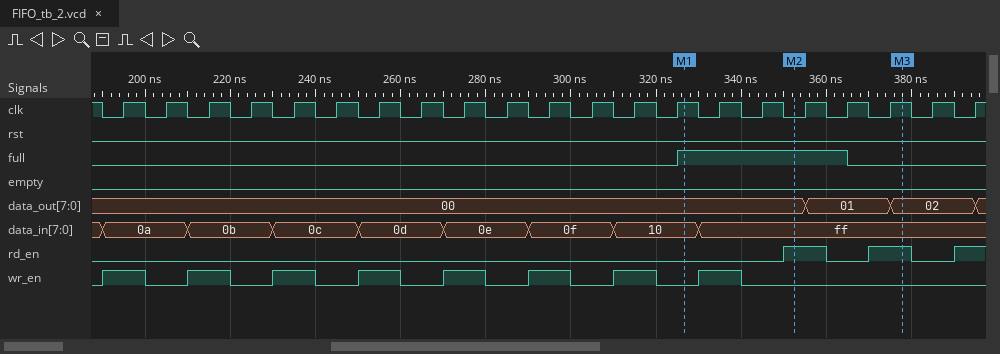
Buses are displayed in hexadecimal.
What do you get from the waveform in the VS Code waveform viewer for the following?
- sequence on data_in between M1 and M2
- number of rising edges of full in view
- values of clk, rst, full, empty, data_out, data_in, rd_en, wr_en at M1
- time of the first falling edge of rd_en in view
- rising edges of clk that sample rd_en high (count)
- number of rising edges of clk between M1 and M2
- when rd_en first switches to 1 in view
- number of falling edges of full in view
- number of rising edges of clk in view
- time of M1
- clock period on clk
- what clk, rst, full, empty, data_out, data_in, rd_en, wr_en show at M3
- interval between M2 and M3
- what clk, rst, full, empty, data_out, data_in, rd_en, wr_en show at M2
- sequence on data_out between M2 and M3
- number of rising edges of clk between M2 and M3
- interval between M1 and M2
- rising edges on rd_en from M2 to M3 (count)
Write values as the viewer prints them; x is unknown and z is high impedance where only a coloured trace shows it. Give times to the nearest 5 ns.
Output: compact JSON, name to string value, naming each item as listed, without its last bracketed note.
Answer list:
{"sequence on data_in between M1 and M2": "10, ff", "number of rising edges of full in view": "1", "values of clk, rst, full, empty, data_out, data_in, rd_en, wr_en at M1": "clk=1, rst=0, full=1, empty=0, data_out=00, data_in=10, rd_en=0, wr_en=0", "time of the first falling edge of rd_en in view": "360 ns", "rising edges of clk that sample rd_en high": "3", "number of rising edges of clk between M1 and M2": "2", "when rd_en first switches to 1 in view": "350 ns", "number of falling edges of full in view": "1", "number of rising edges of clk in view": "21", "time of M1": "325 ns", "clock period on clk": "10 ns", "what clk, rst, full, empty, data_out, data_in, rd_en, wr_en show at M3": "clk=1, rst=0, full=0, empty=0, data_out=02, data_in=ff, rd_en=1, wr_en=0", "interval between M2 and M3": "25 ns", "what clk, rst, full, empty, data_out, data_in, rd_en, wr_en show at M2": "clk=0, rst=0, full=1, empty=0, data_out=00, data_in=ff, rd_en=1, wr_en=0", "sequence on data_out between M2 and M3": "00, 01, 02", "number of rising edges of clk between M2 and M3": "3", "interval between M1 and M2": "25 ns", "rising edges on rd_en from M2 to M3": "1"}
